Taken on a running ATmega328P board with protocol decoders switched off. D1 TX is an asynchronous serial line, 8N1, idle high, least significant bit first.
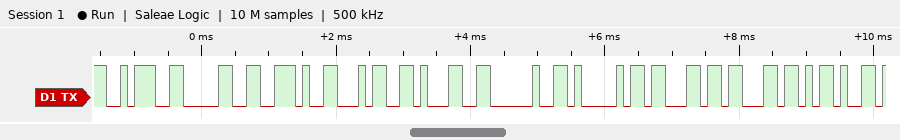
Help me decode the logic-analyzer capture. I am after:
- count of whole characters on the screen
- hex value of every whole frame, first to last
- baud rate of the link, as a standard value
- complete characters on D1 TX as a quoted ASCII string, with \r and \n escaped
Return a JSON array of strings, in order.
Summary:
["10", "3A 30 2E 34 31 20 41 63 63 2D", "9600 baud", "\":0.41 Acc-\""]
